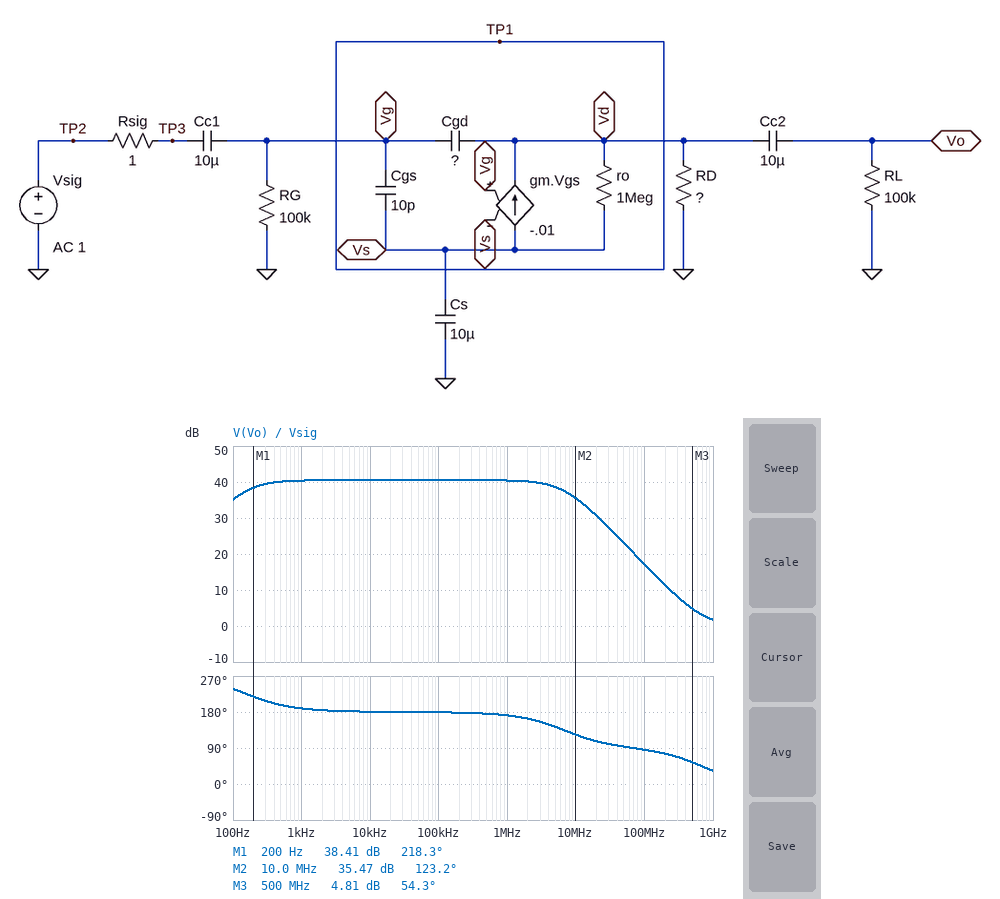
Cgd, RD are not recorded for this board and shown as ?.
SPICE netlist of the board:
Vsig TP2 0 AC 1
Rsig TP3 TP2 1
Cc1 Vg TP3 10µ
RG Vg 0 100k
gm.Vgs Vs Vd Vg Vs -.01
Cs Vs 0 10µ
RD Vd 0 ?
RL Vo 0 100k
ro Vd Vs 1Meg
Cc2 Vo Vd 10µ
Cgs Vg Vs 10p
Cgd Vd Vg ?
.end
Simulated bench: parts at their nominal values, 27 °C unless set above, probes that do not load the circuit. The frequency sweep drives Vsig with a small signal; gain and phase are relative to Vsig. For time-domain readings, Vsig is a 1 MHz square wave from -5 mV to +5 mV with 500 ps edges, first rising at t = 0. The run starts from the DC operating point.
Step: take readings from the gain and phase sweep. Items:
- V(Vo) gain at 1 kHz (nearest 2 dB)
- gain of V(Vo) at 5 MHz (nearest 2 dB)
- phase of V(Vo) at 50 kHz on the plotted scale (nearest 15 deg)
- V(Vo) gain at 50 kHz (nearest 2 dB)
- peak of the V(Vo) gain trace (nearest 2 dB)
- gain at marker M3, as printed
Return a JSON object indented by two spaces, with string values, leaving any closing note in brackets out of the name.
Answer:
{
  "V(Vo) gain at 1 kHz": "40 dB",
  "gain of V(Vo) at 5 MHz": "38 dB",
  "phase of V(Vo) at 50 kHz on the plotted scale": "180 deg",
  "V(Vo) gain at 50 kHz": "40 dB",
  "peak of the V(Vo) gain trace": "40 dB",
  "gain at marker M3, as printed": "4.81 dB"
}
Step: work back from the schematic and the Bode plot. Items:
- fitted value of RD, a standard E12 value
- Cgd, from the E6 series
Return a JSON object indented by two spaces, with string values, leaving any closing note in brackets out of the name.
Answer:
{
  "fitted value of RD, a standard E12 value": "12 kΩ",
  "Cgd, from the E6 series": "2.2 pF"
}
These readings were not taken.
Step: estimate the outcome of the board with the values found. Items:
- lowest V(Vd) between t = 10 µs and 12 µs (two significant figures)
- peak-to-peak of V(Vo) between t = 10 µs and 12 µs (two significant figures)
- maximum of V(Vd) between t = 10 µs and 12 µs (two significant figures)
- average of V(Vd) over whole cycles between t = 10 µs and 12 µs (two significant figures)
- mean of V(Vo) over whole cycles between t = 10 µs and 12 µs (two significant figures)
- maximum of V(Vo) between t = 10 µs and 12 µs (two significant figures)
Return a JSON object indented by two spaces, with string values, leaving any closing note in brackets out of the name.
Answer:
{
  "lowest V(Vd) between t = 10 µs and 12 µs": "-1.1 V",
  "peak-to-peak of V(Vo) between t = 10 µs and 12 µs": "1.1 V",
  "maximum of V(Vd) between t = 10 µs and 12 µs": "8.4 mV",
  "average of V(Vd) over whole cycles between t = 10 µs and 12 µs": "-520 mV",
  "mean of V(Vo) over whole cycles between t = 10 µs and 12 µs": "-520 mV",
  "maximum of V(Vo) between t = 10 µs and 12 µs": "8.4 mV"
}
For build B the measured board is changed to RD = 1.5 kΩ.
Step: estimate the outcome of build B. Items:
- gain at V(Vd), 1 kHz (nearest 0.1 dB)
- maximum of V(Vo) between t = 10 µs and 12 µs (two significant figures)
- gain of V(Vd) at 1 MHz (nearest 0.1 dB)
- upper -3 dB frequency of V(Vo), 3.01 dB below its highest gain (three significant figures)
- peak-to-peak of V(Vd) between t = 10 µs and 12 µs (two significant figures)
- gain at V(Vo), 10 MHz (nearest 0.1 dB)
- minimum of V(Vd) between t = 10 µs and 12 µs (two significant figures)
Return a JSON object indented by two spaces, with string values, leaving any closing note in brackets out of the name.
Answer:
{
  "gain at V(Vd), 1 kHz": "23.3 dB",
  "maximum of V(Vo) between t = 10 µs and 12 µs": "2.9 mV",
  "gain of V(Vd) at 1 MHz": "23.4 dB",
  "upper -3 dB frequency of V(Vo), 3.01 dB below its highest gain": "48.7 MHz",
  "peak-to-peak of V(Vd) between t = 10 µs and 12 µs": "150 mV",
  "gain at V(Vo), 10 MHz": "23.2 dB",
  "minimum of V(Vd) between t = 10 µs and 12 µs": "-150 mV"
}
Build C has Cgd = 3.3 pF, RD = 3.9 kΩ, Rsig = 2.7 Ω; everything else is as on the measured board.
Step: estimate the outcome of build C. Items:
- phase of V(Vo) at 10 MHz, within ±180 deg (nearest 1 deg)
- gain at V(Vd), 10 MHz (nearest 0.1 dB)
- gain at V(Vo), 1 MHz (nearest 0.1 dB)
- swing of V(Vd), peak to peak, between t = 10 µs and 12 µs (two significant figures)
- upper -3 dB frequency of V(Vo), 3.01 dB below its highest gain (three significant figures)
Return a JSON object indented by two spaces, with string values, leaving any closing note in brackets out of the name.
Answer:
{
  "phase of V(Vo) at 10 MHz, within ±180 deg": "140 deg",
  "gain at V(Vd), 10 MHz": "29.3 dB",
  "gain at V(Vo), 1 MHz": "31.4 dB",
  "swing of V(Vd), peak to peak, between t = 10 µs and 12 µs": "380 mV",
  "upper -3 dB frequency of V(Vo), 3.01 dB below its highest gain": "12.6 MHz"
}
